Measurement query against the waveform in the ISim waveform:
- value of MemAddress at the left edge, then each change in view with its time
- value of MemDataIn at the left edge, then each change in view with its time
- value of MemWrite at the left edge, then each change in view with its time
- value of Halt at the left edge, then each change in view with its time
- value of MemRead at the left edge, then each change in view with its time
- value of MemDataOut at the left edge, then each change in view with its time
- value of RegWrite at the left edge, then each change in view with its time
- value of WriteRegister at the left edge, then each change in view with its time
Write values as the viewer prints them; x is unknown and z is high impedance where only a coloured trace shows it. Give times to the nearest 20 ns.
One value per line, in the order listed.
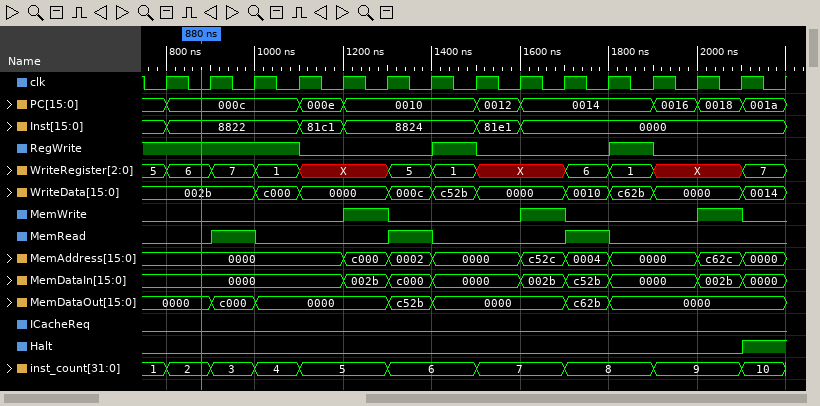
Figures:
0000, c000 at 1200 ns, 0002 at 1300 ns, 0000 at 1400 ns, c52c at 1600 ns, 0004 at 1700 ns, 0000 at 1800 ns, c62c at 2000 ns, 0000 at 2100 ns
0000, 002b at 1200 ns, c000 at 1300 ns, 0000 at 1400 ns, 002b at 1600 ns, c52b at 1700 ns, 0000 at 1800 ns, 002b at 2000 ns, 0000 at 2100 ns
0, 1 at 1200 ns, 0 at 1300 ns, 1 at 1600 ns, 0 at 1700 ns, 1 at 2000 ns, 0 at 2100 ns
0, 1 at 2100 ns
0, 1 at 900 ns, 0 at 1000 ns, 1 at 1300 ns, 0 at 1400 ns, 1 at 1700 ns, 0 at 1800 ns
0000, c000 at 900 ns, 0000 at 1000 ns, c52b at 1300 ns, 0000 at 1400 ns, c62b at 1700 ns, 0000 at 1800 ns
1, 0 at 1100 ns, 1 at 1400 ns, 0 at 1500 ns, 1 at 1800 ns, 0 at 1900 ns
5, 6 at 800 ns, 7 at 900 ns, 1 at 1000 ns, X at 1100 ns, 5 at 1300 ns, 1 at 1400 ns, X at 1500 ns, 6 at 1700 ns, 1 at 1800 ns, X at 1900 ns, 7 at 2100 ns
